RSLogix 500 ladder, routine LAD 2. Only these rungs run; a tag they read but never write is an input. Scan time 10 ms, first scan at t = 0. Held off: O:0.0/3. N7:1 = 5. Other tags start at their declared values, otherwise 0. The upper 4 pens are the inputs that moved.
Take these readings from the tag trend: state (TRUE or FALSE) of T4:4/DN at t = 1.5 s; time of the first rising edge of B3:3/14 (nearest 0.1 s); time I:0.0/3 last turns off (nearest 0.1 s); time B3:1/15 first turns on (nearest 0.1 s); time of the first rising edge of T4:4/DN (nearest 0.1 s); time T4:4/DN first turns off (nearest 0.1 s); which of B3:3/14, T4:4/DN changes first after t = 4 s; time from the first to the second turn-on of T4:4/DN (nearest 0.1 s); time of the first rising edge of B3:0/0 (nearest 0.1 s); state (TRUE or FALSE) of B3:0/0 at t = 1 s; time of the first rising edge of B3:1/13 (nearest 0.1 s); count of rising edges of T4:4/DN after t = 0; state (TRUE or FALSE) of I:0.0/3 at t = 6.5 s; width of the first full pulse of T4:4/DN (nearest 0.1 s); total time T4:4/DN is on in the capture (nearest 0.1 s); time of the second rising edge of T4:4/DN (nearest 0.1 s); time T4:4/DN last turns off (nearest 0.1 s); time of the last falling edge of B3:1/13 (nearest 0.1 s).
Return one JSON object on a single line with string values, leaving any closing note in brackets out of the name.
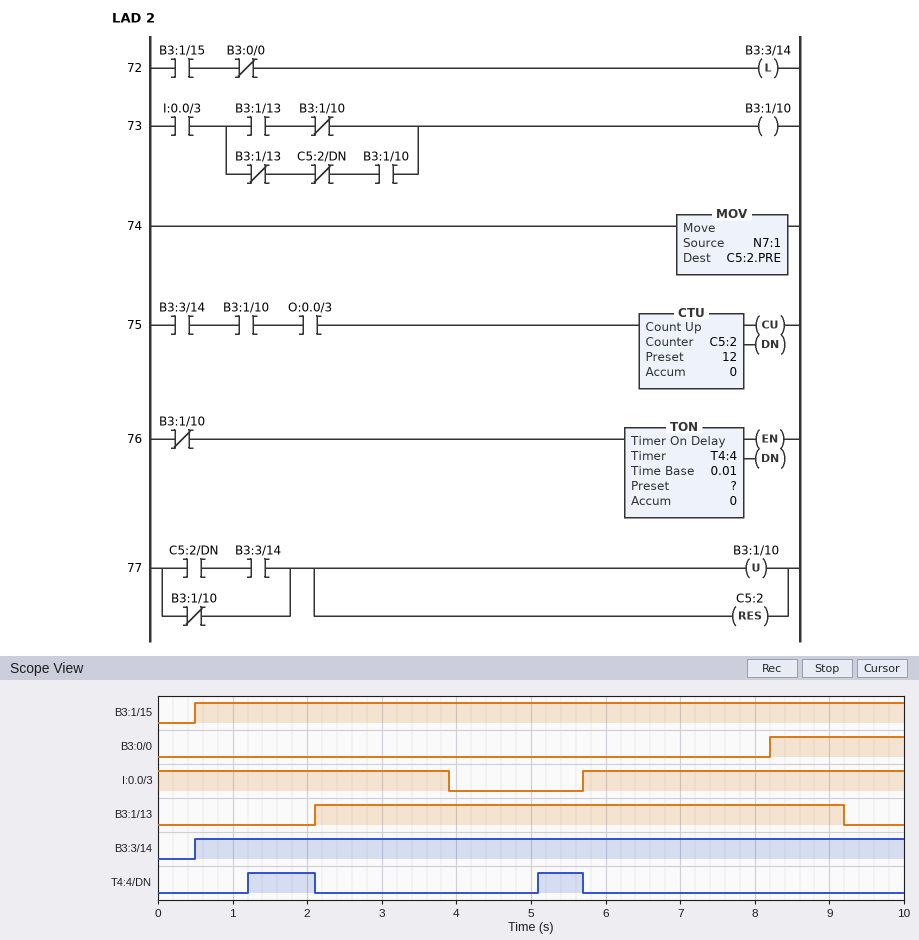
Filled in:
{"state (TRUE or FALSE) of T4:4/DN at t = 1.5 s": "TRUE", "time of the first rising edge of B3:3/14": "0.5 s", "time I:0.0/3 last turns off": "3.9 s", "time B3:1/15 first turns on": "0.5 s", "time of the first rising edge of T4:4/DN": "1.2 s", "time T4:4/DN first turns off": "2.1 s", "which of B3:3/14, T4:4/DN changes first after t = 4 s": "T4:4/DN", "time from the first to the second turn-on of T4:4/DN": "3.9 s", "time of the first rising edge of B3:0/0": "8.2 s", "state (TRUE or FALSE) of B3:0/0 at t = 1 s": "FALSE", "time of the first rising edge of B3:1/13": "2.1 s", "count of rising edges of T4:4/DN after t = 0": "2", "state (TRUE or FALSE) of I:0.0/3 at t = 6.5 s": "TRUE", "width of the first full pulse of T4:4/DN": "0.9 s", "total time T4:4/DN is on in the capture": "1.5 s", "time of the second rising edge of T4:4/DN": "5.1 s", "time T4:4/DN last turns off": "5.7 s", "time of the last falling edge of B3:1/13": "9.2 s"}
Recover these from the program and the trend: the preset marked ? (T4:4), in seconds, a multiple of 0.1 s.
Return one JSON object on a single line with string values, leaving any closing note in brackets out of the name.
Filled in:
{"the preset marked ? (T4:4), in seconds, a multiple of 0.1 s": "1.2 s"}
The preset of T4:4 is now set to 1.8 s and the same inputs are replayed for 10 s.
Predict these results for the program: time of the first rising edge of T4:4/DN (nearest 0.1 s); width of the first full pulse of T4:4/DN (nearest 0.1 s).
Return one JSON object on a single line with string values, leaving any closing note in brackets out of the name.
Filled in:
{"time of the first rising edge of T4:4/DN": "1.8 s", "width of the first full pulse of T4:4/DN": "0.3 s"}
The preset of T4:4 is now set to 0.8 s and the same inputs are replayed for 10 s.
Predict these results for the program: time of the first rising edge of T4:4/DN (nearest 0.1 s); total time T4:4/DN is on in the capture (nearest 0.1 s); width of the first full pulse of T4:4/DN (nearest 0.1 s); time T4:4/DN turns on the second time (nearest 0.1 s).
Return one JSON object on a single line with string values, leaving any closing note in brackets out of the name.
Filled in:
{"time of the first rising edge of T4:4/DN": "0.8 s", "total time T4:4/DN is on in the capture": "2.3 s", "width of the first full pulse of T4:4/DN": "1.3 s", "time T4:4/DN turns on the second time": "4.7 s"}
